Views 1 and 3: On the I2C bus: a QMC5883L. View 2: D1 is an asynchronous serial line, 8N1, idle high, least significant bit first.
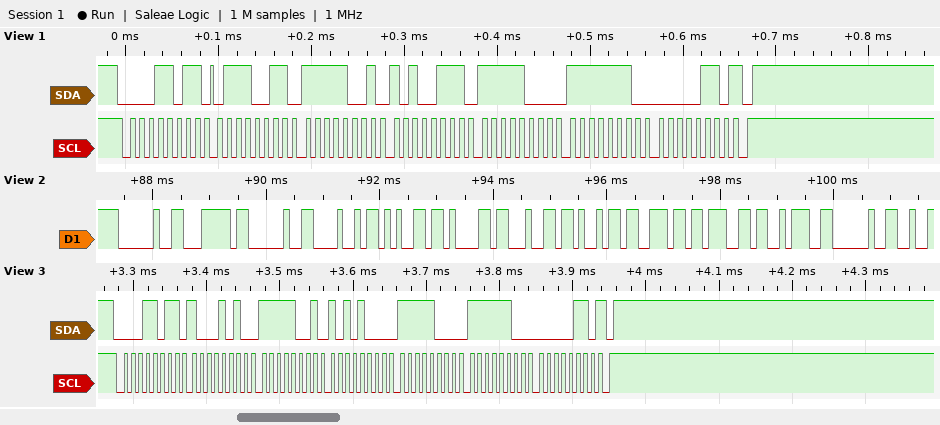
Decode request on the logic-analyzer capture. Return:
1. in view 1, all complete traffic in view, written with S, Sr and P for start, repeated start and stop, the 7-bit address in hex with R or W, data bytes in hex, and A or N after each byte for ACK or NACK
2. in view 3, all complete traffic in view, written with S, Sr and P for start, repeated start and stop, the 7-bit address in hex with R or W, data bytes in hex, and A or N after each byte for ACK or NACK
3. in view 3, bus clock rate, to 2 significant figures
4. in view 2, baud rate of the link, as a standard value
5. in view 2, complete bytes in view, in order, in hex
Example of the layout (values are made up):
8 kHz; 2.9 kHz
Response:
S 0DR A 73 A F9 A A7 A F8 A FE A 06 N P; S 0DR A 8A A F9 A A8 A F8 A FC A 06 N P; 100 kHz; 9600 baud; 20 7C 20 48 65 61 64 69 6E 67 3A 20
